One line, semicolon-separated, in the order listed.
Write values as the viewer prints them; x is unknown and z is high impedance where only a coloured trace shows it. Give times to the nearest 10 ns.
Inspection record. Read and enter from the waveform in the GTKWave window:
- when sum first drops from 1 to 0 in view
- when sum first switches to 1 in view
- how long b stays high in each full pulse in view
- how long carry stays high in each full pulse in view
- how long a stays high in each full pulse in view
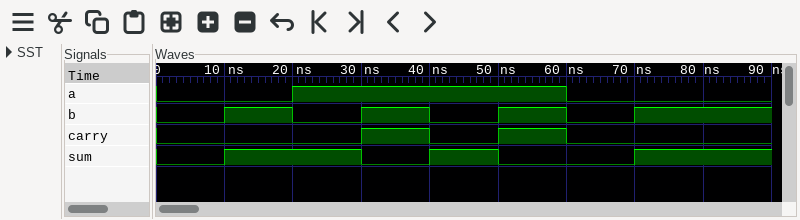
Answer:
30 ns; 10 ns; 10 ns, 10 ns, 10 ns; 10 ns, 10 ns; 40 ns
